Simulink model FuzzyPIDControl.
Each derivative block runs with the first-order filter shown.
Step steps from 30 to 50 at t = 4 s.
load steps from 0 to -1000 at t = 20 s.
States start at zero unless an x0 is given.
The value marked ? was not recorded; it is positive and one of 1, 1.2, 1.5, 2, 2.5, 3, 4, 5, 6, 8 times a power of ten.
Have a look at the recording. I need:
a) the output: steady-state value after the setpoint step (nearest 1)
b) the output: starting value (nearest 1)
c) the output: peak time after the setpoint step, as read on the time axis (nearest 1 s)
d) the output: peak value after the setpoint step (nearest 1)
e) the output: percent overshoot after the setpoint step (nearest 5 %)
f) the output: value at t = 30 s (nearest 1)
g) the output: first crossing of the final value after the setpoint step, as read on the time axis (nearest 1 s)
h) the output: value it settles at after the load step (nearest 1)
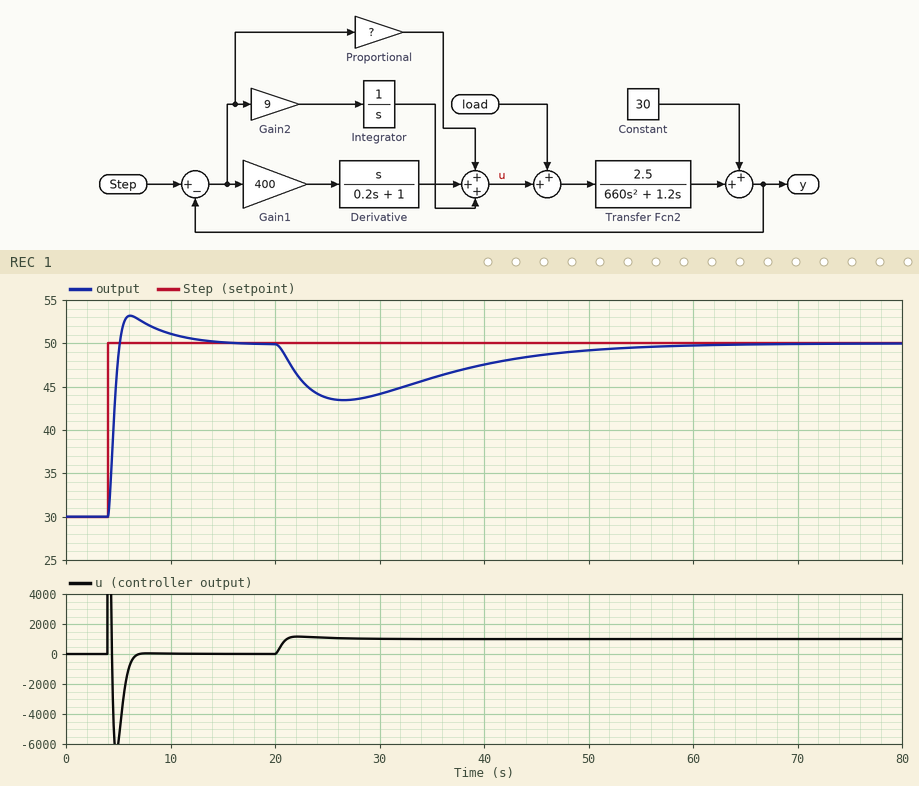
50
30
6 s
53
15 %
44
5 s
50
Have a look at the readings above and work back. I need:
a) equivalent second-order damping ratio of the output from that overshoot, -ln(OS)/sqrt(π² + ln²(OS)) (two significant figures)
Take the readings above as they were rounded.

0.52
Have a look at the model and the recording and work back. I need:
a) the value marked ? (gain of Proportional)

120
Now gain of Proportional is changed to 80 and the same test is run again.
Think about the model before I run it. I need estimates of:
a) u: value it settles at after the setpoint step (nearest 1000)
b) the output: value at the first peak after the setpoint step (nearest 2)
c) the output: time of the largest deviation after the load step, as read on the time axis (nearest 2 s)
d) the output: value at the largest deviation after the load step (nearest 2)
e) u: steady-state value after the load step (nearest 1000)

0
52
28 s
42
1000
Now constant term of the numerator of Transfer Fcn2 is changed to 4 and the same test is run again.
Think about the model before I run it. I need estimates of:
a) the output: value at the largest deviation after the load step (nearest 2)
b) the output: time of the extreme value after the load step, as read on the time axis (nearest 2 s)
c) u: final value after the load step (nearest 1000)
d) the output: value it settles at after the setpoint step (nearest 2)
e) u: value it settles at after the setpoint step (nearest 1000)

44
26 s
1000
50
0
